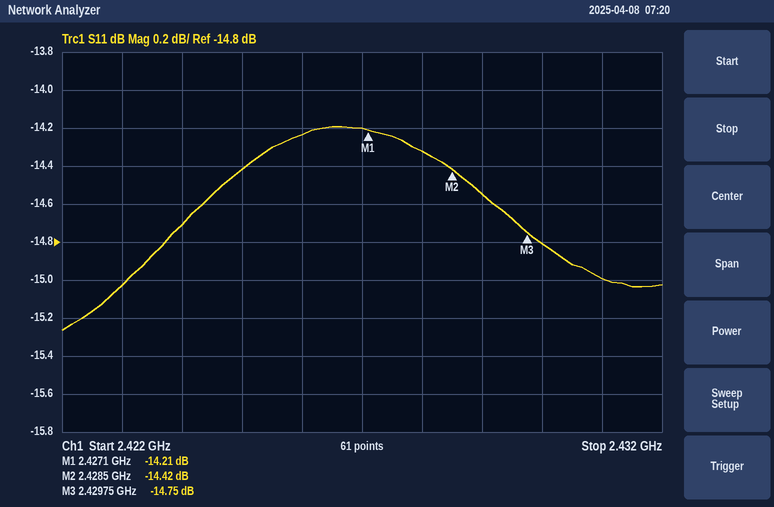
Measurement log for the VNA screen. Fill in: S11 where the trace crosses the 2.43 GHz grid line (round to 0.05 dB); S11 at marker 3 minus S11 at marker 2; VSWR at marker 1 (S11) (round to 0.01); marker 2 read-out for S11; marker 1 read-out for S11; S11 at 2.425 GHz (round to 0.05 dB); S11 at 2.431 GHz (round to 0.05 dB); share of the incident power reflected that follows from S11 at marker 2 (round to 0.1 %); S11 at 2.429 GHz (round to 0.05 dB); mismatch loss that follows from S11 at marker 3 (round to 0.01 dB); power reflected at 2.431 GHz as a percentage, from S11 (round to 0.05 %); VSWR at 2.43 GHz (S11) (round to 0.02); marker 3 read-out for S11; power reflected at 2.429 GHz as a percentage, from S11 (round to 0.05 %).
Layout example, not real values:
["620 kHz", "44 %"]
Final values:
["-14.80 dB", "-0.33 dB", "1.48", "-14.42 dB", "-14.21 dB", "-14.40 dB", "-15.00 dB", "3.6 %", "-14.55 dB", "0.15 dB", "3.15 %", "1.44", "-14.75 dB", "3.50 %"]
